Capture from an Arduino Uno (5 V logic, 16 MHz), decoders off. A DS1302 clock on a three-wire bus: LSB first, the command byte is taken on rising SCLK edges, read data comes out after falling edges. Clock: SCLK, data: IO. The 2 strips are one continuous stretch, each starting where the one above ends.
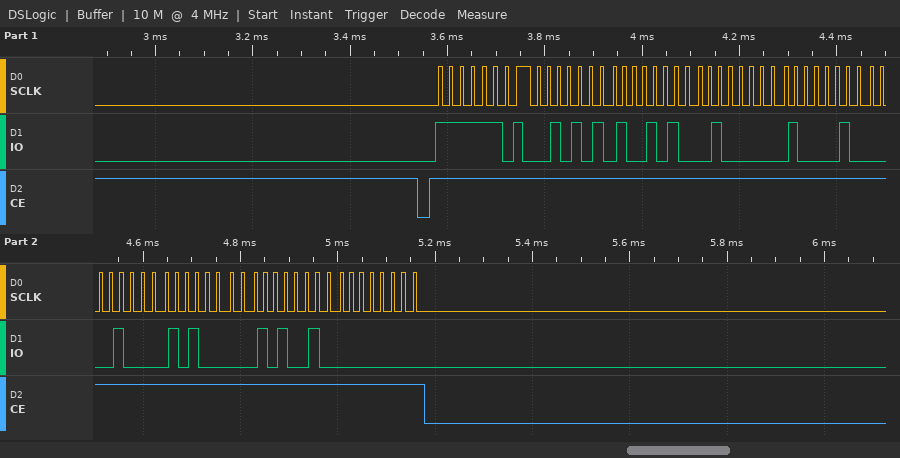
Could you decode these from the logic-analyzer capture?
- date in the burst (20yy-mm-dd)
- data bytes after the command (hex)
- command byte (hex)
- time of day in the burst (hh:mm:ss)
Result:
2025-08-21
54 29 02 21 08 05 25 00
0xBF
02:29:54
